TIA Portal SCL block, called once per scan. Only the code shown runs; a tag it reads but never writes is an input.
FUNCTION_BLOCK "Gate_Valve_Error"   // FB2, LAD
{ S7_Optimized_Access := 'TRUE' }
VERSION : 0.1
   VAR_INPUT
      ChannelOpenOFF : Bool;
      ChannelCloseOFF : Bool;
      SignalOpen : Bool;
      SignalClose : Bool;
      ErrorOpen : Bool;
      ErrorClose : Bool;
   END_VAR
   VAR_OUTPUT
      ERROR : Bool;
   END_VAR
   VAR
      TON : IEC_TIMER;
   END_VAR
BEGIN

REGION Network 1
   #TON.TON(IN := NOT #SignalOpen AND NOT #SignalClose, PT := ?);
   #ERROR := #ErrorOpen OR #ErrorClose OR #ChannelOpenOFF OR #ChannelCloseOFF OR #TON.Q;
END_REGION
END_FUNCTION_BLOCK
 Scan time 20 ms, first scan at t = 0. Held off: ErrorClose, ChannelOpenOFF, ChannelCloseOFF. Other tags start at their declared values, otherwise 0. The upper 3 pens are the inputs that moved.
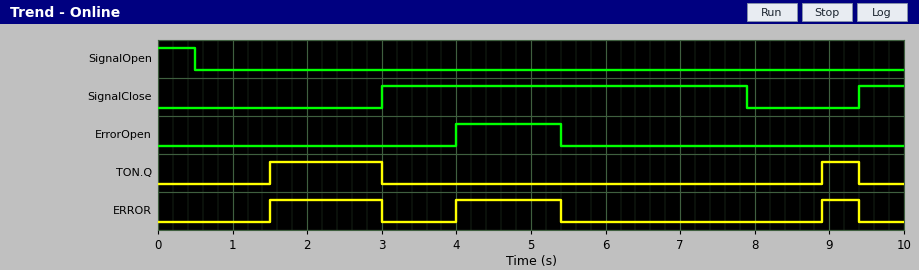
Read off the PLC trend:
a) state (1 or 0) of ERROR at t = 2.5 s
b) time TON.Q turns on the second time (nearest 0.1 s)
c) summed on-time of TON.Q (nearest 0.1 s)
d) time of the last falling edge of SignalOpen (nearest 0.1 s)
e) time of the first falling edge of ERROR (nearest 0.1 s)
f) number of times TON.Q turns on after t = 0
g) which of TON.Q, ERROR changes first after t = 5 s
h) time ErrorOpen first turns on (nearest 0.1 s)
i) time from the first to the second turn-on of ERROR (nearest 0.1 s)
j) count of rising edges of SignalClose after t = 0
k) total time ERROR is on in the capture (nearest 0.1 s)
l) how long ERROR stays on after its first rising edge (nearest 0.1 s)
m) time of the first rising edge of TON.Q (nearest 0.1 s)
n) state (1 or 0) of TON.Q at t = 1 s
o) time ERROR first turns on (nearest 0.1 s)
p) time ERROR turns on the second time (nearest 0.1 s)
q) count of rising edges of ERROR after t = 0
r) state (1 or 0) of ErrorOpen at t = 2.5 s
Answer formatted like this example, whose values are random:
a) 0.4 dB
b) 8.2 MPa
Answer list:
a) 1
b) 8.9 s
c) 2.0 s
d) 0.5 s
e) 3.0 s
f) 2
g) ERROR
h) 4.0 s
i) 2.5 s
j) 2
k) 3.4 s
l) 1.5 s
m) 1.5 s
n) 0
o) 1.5 s
p) 4.0 s
q) 3
r) 0
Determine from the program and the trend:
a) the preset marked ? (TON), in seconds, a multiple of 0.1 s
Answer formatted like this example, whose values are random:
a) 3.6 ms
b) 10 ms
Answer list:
a) 1.0 s
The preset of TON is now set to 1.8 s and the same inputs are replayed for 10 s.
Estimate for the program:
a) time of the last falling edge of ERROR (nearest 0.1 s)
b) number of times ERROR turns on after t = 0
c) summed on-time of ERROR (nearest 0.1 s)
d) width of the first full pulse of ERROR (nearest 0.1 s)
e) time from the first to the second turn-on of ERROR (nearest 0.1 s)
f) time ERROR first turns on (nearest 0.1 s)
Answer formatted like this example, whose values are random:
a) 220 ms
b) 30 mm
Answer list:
a) 5.4 s
b) 2
c) 2.1 s
d) 0.7 s
e) 1.7 s
f) 2.3 s
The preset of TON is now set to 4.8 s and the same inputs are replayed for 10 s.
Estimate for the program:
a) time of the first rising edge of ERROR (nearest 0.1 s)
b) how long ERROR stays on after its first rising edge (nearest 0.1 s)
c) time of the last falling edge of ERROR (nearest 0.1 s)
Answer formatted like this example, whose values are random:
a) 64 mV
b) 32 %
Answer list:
a) 4.0 s
b) 1.4 s
c) 5.4 s
